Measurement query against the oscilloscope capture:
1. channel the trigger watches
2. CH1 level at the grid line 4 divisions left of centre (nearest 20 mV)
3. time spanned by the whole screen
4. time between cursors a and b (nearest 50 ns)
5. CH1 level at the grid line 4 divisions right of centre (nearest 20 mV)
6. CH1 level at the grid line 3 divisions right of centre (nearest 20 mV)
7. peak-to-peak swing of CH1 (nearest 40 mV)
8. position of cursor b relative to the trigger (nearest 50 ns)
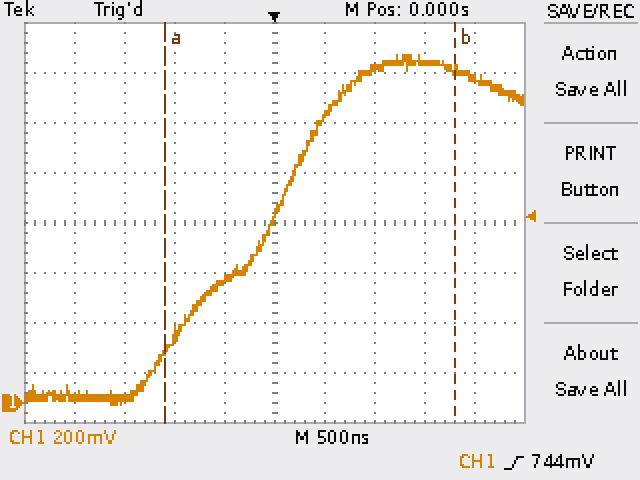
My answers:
CH1
20 mV
5 µs
2.90 µs
1.30 V
1.36 V
1.40 V
+1.80 µs
